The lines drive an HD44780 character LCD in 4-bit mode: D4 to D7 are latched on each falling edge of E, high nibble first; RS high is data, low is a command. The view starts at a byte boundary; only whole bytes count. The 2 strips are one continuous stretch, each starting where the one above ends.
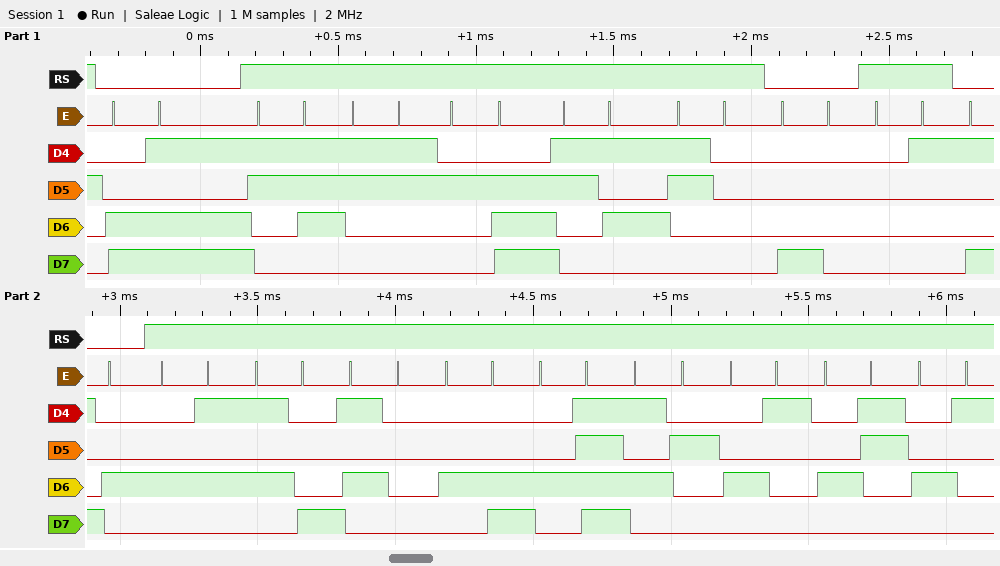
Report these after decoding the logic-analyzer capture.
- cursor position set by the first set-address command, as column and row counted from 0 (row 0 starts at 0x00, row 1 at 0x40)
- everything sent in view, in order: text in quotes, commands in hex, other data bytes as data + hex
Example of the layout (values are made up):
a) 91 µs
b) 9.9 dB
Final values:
a) column 13, row 1
b) 0xCD "73.50" 0x80 data 01 0x94 "EXPLORACA"
